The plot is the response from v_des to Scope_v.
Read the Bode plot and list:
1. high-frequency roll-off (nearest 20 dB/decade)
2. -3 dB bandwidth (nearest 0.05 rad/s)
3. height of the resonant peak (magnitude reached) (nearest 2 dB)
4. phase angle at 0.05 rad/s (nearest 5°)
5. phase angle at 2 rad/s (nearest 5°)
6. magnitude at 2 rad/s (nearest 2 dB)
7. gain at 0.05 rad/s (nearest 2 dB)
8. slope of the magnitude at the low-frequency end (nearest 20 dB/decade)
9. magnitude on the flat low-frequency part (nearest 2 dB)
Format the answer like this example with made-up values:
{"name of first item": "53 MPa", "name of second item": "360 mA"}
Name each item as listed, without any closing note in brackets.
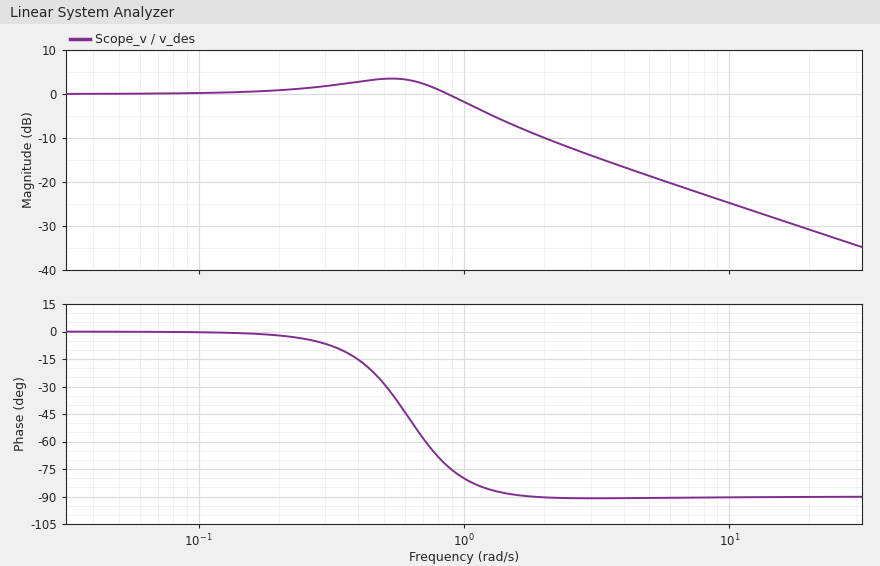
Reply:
{"high-frequency roll-off": "-20 dB/decade", "-3 dB bandwidth": "1.10 rad/s", "height of the resonant peak (magnitude reached)": "4 dB", "phase angle at 0.05 rad/s": "0°", "phase angle at 2 rad/s": "-90°", "magnitude at 2 rad/s": "-10 dB", "gain at 0.05 rad/s": "0 dB", "slope of the magnitude at the low-frequency end": "0 dB/decade", "magnitude on the flat low-frequency part": "0 dB"}
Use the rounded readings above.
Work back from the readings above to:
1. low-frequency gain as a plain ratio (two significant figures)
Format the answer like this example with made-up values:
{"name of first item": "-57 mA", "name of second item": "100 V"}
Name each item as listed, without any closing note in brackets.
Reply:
{"low-frequency gain as a plain ratio": "1.0"}
